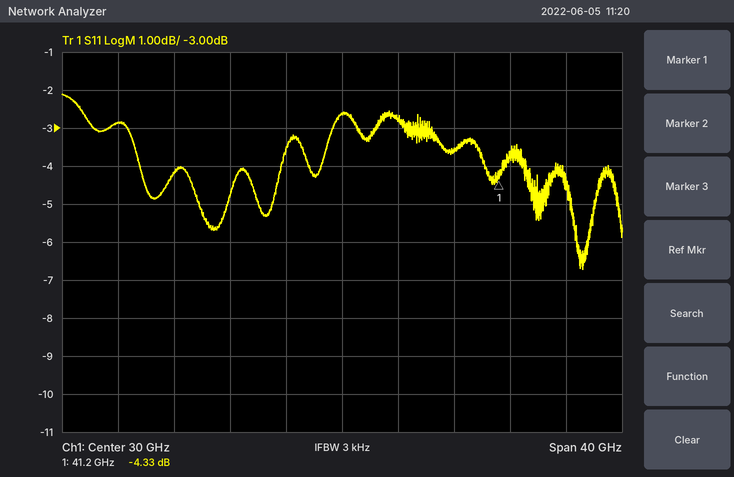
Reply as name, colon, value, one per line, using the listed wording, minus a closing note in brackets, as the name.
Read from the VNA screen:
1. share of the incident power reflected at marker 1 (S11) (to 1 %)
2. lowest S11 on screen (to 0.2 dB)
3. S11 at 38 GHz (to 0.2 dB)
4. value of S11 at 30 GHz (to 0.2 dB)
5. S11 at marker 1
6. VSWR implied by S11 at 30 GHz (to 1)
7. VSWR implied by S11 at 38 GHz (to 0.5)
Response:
share of the incident power reflected at marker 1 (S11): 37 %
lowest S11 on screen: -6.8 dB
S11 at 38 GHz: -3.6 dB
value of S11 at 30 GHz: -2.6 dB
S11 at marker 1: -4.33 dB
VSWR implied by S11 at 30 GHz: 7
VSWR implied by S11 at 38 GHz: 5.0
